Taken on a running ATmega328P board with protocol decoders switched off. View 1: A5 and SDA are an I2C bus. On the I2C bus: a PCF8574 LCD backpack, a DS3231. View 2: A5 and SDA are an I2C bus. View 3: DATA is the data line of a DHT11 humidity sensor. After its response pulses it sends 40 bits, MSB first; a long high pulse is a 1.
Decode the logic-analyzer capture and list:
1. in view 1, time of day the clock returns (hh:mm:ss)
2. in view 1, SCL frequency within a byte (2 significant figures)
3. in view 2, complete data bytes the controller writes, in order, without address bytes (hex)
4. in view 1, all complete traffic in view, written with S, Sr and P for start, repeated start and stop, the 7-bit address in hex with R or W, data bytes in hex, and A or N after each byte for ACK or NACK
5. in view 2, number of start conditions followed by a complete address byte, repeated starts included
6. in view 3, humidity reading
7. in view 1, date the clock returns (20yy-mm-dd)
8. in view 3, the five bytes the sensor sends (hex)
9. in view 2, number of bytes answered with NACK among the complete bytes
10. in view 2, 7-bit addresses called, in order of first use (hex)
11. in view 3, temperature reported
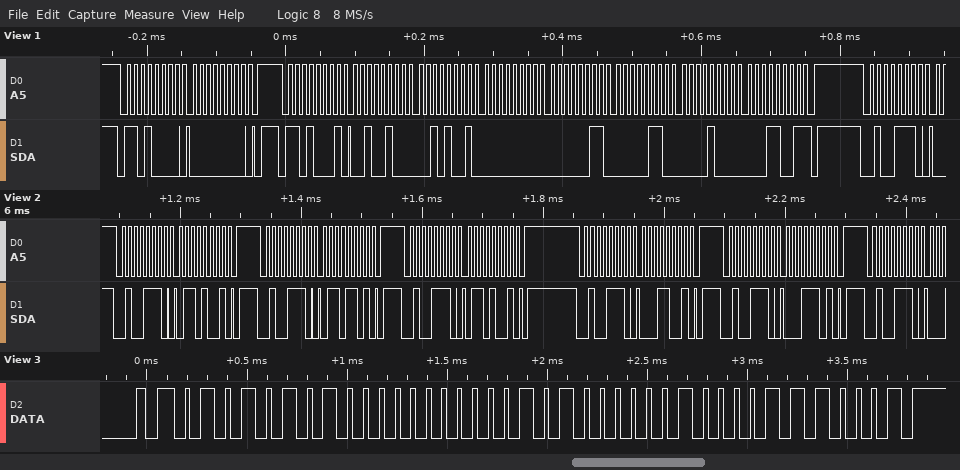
00:29:24
100 kHz
69 6D 69 19 1D
S 68W A 00 A P S 68R A 24 A 29 A 00 A 03 A 06 A 08 A 19 N P S 27W A
6
85 %
2019-08-06
55 00 14 08 71
0
0x27
20.8 °C
